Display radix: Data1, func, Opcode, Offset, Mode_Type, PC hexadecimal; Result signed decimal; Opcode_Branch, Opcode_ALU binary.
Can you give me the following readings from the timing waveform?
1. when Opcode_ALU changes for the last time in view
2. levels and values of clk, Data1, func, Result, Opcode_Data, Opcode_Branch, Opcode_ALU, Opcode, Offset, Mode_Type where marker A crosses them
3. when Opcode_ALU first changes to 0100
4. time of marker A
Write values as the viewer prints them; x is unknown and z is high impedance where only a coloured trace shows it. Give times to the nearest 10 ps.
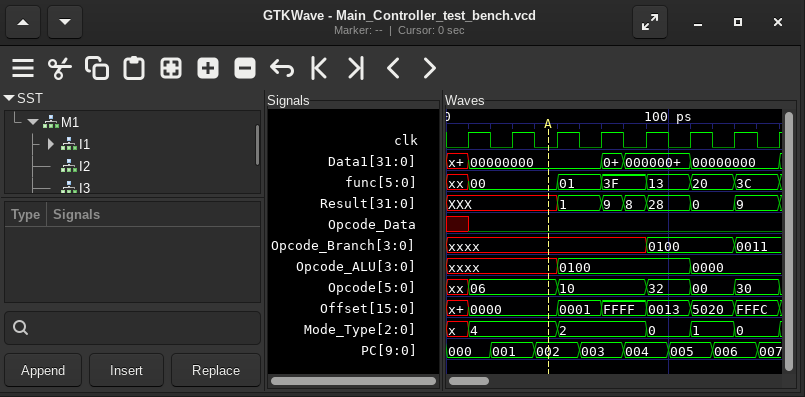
110 ps
clk=0, Data1=00000000, func=00, Result=XXX, Opcode_Data=0, Opcode_Branch=xxxx, Opcode_ALU=xxxx, Opcode=06, Offset=0000, Mode_Type=4
50 ps
50 ps
